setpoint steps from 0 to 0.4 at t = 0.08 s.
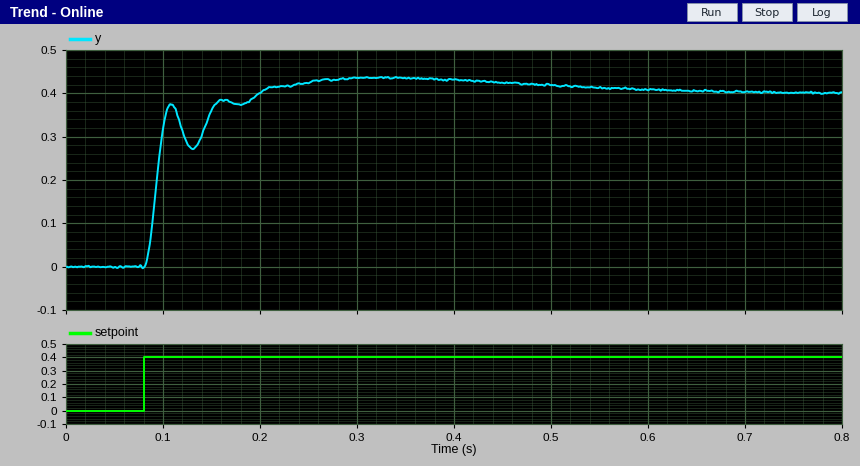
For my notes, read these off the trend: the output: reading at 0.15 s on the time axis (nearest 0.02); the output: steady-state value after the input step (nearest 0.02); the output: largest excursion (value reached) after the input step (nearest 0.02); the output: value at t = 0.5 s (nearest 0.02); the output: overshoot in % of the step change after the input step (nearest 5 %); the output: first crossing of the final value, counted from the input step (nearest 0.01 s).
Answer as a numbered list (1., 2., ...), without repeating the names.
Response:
1. 0.36
2. 0.40
3. 0.44
4. 0.42
5. 10 %
6. 0.12 s
